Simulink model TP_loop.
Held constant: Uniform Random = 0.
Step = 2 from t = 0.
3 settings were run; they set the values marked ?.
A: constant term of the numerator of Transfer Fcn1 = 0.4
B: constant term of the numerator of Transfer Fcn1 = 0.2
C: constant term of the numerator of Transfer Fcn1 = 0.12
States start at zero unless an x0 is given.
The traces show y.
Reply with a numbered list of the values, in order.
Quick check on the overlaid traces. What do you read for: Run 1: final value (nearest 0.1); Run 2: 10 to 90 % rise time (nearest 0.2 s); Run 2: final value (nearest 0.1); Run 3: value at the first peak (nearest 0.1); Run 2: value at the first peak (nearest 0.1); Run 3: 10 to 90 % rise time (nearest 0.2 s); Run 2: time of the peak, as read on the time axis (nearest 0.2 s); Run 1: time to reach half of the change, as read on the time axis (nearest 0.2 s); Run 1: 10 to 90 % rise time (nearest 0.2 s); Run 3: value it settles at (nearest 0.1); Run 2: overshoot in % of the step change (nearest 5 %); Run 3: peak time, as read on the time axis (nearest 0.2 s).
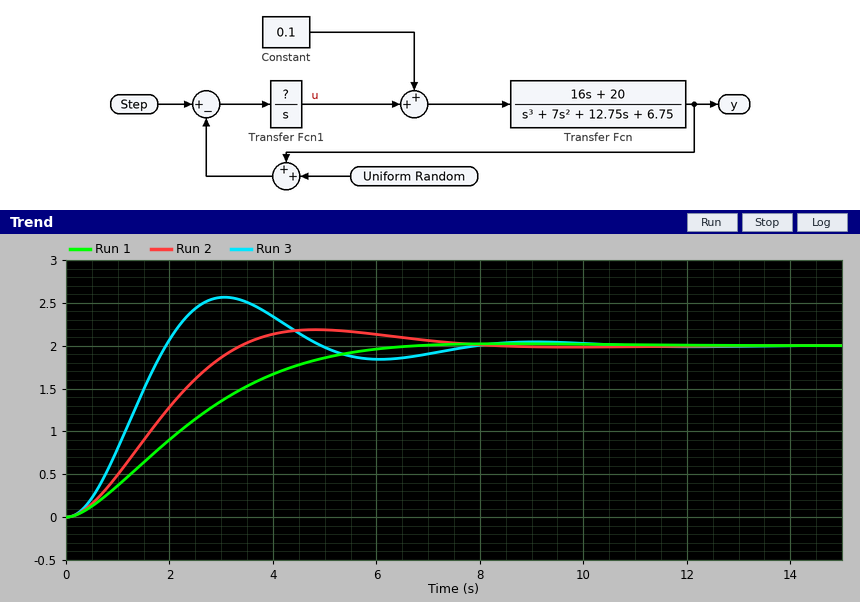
1. 2.0
2. 2.2 s
3. 2.0
4. 2.6
5. 2.2
6. 1.2 s
7. 4.8 s
8. 2.2 s
9. 4.0 s
10. 2.0
11. 10 %
12. 3.0 s
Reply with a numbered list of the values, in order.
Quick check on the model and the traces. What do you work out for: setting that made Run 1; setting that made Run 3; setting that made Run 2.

1. C
2. A
3. B
